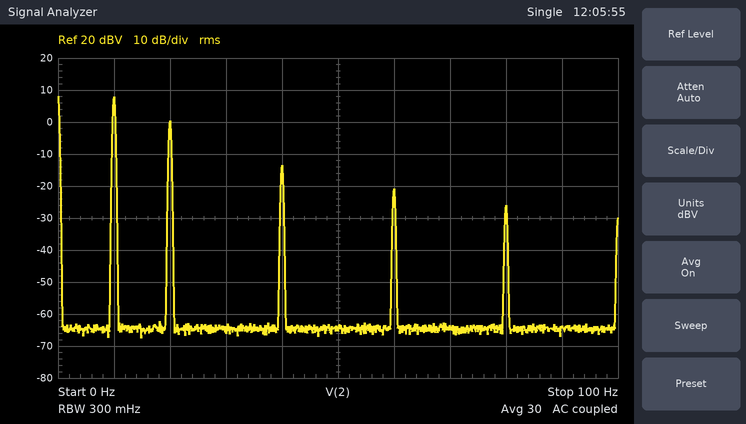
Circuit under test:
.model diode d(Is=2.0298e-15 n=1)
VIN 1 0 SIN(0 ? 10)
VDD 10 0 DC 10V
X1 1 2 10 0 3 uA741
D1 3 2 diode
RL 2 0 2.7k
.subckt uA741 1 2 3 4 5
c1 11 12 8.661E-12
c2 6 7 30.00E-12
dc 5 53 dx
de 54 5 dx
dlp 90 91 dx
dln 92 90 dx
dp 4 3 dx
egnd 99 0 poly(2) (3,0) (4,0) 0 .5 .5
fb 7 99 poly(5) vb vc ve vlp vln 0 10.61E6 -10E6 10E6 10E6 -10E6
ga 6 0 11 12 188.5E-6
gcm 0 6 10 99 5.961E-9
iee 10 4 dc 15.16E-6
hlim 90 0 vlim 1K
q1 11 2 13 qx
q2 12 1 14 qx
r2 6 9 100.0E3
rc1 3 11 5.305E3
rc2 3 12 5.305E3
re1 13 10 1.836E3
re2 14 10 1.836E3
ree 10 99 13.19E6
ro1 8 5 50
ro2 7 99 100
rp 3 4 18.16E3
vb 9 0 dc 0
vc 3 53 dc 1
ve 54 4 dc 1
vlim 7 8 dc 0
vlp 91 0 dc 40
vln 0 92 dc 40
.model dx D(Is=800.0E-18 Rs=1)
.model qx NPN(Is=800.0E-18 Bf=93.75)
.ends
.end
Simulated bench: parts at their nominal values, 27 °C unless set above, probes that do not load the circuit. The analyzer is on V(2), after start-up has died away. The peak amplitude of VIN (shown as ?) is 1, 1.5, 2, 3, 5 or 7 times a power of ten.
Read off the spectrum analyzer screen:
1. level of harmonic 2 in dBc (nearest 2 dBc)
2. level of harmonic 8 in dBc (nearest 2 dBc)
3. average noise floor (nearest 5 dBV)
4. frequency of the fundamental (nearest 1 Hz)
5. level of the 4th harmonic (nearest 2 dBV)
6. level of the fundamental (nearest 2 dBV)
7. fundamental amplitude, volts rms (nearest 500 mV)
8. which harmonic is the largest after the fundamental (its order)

-8 dBc
-34 dBc
-65 dBV
10 Hz
-14 dBV
8 dBV
2.5 V
2
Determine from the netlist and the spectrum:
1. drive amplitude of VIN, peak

7 V
